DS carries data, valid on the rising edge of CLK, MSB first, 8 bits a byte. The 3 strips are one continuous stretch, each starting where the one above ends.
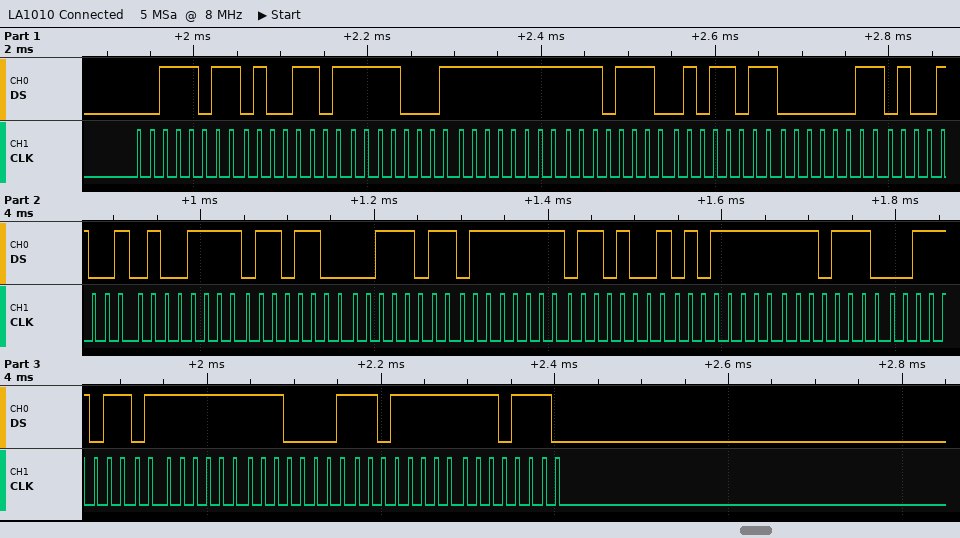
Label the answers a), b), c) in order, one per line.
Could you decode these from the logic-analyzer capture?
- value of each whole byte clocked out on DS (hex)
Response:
a) 3B 4D F1 FF EE 5B 03 49 4F 6C 3B 7F 69 5F EE 3B 7F E1 DF EE
